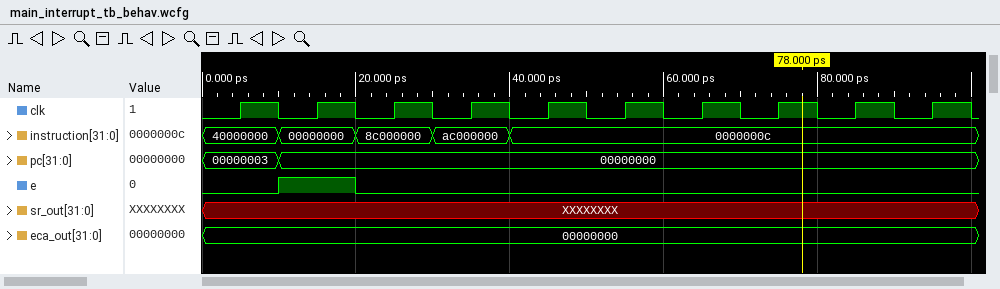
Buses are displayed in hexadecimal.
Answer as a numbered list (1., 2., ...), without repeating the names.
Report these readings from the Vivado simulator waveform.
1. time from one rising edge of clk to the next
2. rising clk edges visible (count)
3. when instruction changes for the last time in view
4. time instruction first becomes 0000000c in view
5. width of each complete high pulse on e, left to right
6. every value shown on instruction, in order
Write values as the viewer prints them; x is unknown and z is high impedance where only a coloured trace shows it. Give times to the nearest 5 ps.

1. 10 ps
2. 10
3. 40 ps
4. 40 ps
5. 10 ps
6. 40000000, 00000000, 8c000000, ac000000, 0000000c
